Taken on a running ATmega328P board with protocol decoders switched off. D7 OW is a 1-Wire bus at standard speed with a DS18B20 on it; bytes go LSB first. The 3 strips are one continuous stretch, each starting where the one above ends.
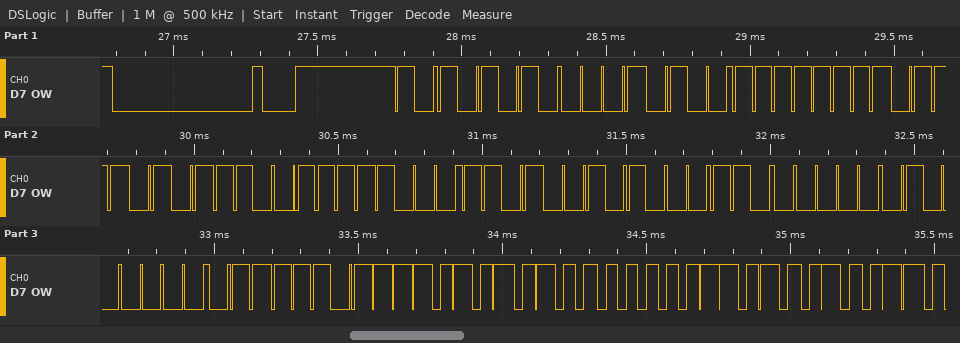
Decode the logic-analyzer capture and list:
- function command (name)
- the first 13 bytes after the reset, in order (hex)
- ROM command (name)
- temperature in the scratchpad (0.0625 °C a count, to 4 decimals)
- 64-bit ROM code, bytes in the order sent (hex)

Read Scratchpad
55 28 FF AE F3 B1 14 03 02 BE 57 01 4B
Match ROM
21.4375 °C
28 FF AE F3 B1 14 03 02
